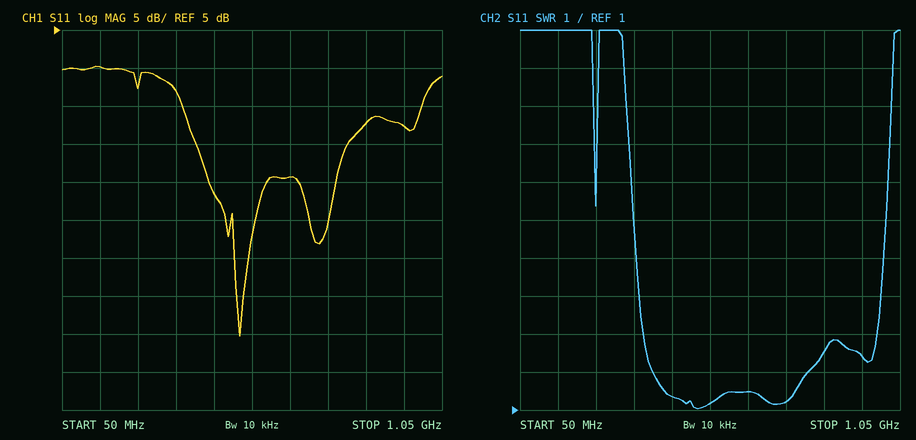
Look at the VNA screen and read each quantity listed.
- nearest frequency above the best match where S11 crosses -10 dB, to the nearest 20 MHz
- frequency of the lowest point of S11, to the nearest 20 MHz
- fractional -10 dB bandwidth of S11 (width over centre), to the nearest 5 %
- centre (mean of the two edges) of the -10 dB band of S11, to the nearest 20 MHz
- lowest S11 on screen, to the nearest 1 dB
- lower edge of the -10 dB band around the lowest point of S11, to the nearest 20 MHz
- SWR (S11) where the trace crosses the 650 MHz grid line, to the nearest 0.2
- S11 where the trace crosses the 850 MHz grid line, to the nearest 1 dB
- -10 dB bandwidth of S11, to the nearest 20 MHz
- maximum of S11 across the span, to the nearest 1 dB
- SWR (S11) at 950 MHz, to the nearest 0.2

800 MHz
520 MHz
65 %
600 MHz
-35 dB
400 MHz
1.4
-7 dB
400 MHz
0 dB
2.4
